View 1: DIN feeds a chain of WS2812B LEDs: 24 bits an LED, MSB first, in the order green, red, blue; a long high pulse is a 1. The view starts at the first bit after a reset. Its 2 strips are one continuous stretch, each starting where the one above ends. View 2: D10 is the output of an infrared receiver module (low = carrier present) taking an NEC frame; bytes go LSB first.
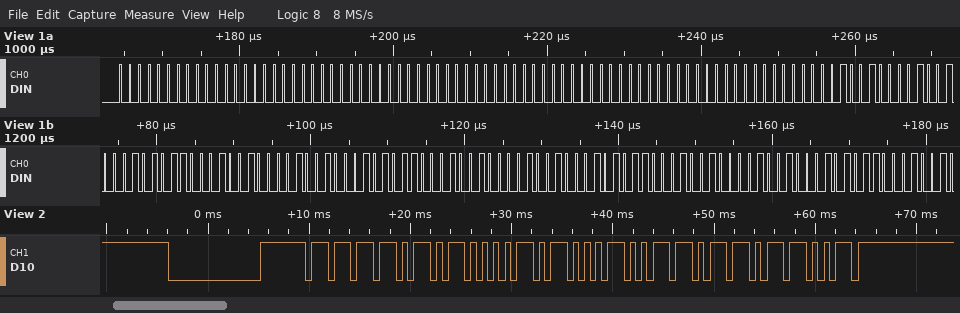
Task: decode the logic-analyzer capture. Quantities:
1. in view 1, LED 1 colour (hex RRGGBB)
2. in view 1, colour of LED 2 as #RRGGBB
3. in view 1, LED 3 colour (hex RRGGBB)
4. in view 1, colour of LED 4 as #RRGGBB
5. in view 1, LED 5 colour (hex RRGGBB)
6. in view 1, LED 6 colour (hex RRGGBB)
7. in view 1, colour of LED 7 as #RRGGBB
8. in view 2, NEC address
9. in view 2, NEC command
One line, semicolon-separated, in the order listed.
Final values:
#000000; #000000; #000000; #12122B; #12122B; #12122B; #12122B; 0xAF; 0x64
